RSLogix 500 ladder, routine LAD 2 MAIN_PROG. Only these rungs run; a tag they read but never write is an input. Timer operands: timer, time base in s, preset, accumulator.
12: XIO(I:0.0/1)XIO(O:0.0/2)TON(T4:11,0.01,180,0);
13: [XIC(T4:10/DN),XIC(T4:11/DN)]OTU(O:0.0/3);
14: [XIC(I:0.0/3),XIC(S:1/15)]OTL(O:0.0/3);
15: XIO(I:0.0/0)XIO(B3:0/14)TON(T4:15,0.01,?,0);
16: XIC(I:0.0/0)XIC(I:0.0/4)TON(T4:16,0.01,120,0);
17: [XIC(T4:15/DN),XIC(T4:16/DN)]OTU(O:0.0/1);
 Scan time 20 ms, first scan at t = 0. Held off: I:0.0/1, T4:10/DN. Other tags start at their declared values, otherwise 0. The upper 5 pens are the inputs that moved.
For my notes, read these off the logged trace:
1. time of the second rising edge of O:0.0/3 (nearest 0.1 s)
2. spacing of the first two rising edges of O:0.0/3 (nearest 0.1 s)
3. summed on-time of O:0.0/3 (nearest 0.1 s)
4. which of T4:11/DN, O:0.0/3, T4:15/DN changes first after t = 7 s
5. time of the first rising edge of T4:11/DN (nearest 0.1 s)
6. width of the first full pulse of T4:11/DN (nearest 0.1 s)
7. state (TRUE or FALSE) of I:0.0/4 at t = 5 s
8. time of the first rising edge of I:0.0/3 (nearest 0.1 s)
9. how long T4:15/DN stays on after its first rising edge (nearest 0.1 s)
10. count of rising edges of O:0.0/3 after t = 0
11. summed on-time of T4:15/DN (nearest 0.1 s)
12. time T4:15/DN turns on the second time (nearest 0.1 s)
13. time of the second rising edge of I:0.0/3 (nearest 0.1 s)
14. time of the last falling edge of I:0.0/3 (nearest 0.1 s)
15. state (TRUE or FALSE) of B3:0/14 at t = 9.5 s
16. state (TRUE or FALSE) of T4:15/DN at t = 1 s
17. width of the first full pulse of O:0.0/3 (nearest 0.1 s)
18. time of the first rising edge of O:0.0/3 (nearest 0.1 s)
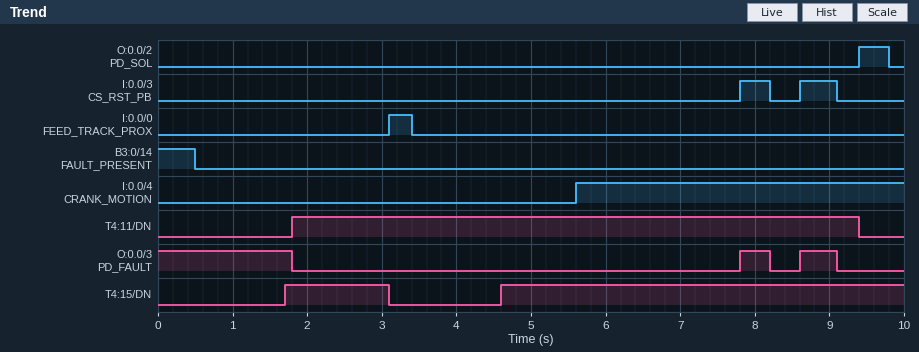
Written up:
8.6 s
0.8 s
2.7 s
O:0.0/3
1.8 s
7.6 s
FALSE
7.8 s
1.4 s
2
6.8 s
4.6 s
8.6 s
9.1 s
FALSE
FALSE
0.4 s
7.8 s
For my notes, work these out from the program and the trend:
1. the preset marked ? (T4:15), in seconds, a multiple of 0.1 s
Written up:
1.2 s
